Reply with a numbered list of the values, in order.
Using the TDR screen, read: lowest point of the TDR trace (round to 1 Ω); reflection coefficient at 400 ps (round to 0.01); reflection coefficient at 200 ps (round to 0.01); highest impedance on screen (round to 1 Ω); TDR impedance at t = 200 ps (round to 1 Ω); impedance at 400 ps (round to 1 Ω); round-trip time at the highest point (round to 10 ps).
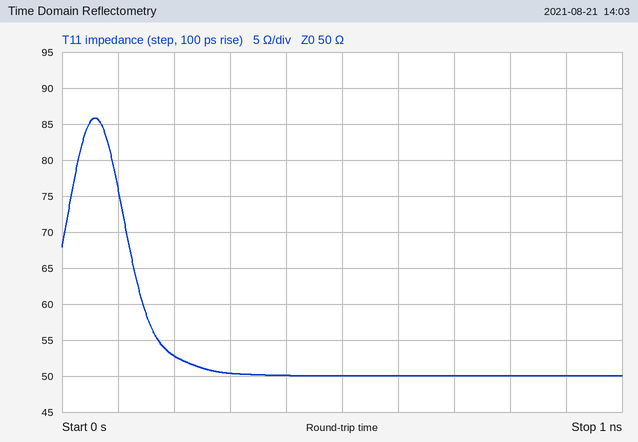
1. 50 Ω
2. 0.00
3. +0.03
4. 86 Ω
5. 53 Ω
6. 50 Ω
7. 60 ps
